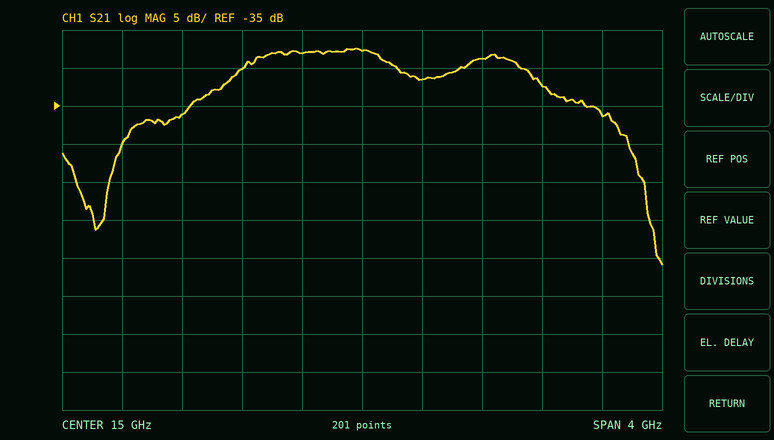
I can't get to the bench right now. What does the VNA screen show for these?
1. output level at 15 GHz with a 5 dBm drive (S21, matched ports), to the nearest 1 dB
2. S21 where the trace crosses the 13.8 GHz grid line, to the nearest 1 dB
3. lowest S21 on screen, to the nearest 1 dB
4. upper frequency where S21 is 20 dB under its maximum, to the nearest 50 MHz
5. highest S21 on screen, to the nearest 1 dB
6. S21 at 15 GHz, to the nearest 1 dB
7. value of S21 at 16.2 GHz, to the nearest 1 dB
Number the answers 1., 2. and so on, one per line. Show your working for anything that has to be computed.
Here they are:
1. 5 dBm + (-28 dB) = -23 dBm
2. -36 dB
3. -56 dB
4. 16.90 GHz
5. -27 dB
6. -28 dB
7. -32 dB
